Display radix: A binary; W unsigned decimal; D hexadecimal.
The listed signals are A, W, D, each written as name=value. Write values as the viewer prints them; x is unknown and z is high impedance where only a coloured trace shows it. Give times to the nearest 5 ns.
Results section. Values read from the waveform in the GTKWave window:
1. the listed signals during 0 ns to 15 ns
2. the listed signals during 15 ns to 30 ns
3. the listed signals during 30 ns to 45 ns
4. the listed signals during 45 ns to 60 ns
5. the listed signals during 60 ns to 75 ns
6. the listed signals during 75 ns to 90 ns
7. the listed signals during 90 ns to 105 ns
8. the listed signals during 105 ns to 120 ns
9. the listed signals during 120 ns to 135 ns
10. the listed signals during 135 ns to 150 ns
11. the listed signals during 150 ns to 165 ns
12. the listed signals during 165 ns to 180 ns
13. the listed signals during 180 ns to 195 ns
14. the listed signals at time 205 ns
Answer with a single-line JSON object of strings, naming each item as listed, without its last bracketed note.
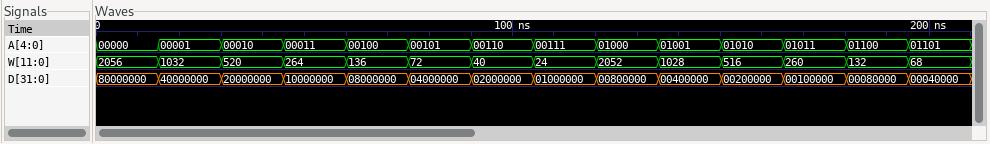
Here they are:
{"the listed signals during 0 ns to 15 ns": "A=00000, W=2056, D=80000000", "the listed signals during 15 ns to 30 ns": "A=00001, W=1032, D=40000000", "the listed signals during 30 ns to 45 ns": "A=00010, W=520, D=20000000", "the listed signals during 45 ns to 60 ns": "A=00011, W=264, D=10000000", "the listed signals during 60 ns to 75 ns": "A=00100, W=136, D=08000000", "the listed signals during 75 ns to 90 ns": "A=00101, W=72, D=04000000", "the listed signals during 90 ns to 105 ns": "A=00110, W=40, D=02000000", "the listed signals during 105 ns to 120 ns": "A=00111, W=24, D=01000000", "the listed signals during 120 ns to 135 ns": "A=01000, W=2052, D=00800000", "the listed signals during 135 ns to 150 ns": "A=01001, W=1028, D=00400000", "the listed signals during 150 ns to 165 ns": "A=01010, W=516, D=00200000", "the listed signals during 165 ns to 180 ns": "A=01011, W=260, D=00100000", "the listed signals during 180 ns to 195 ns": "A=01100, W=132, D=00080000", "the listed signals at time 205 ns": "A=01101, W=68, D=00040000"}
